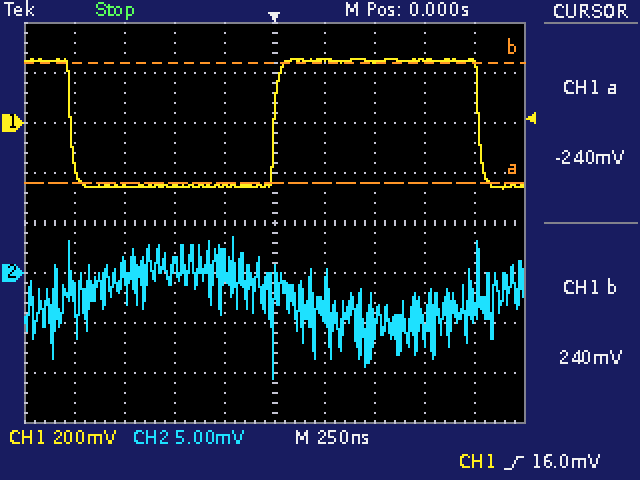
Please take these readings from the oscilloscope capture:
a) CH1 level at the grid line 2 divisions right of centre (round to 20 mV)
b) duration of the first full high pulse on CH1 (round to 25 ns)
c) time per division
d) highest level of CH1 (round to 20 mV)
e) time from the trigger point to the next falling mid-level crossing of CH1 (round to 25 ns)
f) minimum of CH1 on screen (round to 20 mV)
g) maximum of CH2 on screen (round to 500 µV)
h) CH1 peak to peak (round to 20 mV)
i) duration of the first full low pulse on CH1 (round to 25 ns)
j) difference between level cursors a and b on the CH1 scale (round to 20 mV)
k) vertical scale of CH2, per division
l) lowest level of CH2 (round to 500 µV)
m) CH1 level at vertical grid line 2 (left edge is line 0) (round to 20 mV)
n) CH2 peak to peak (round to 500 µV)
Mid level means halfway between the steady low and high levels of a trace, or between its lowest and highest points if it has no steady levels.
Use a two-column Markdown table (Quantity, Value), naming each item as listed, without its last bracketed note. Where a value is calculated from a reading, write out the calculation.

| Quantity | Value |
|---|---|
| CH1 level at the grid line 2 divisions right of centre | 240 mV |
| duration of the first full high pulse on CH1 | 1.025 µs |
| time per division | 250 ns |
| highest level of CH1 | 260 mV |
| time from the trigger point to the next falling mid-level crossing of CH1 | 1.025 µs |
| minimum of CH1 on screen | -260 mV |
| maximum of CH2 on screen | 3.5 mV |
| CH1 peak to peak | 260 mV − (-260 mV) = 520 mV |
| duration of the first full low pulse on CH1 | 1.025 µs |
| difference between level cursors a and b on the CH1 scale | 480 mV |
| vertical scale of CH2, per division | 5 mV |
| lowest level of CH2 | -10.5 mV |
| CH1 level at vertical grid line 2 (left edge is line 0) | -260 mV |
| CH2 peak to peak | 3.5 mV − (-10.5 mV) = 14.0 mV |
